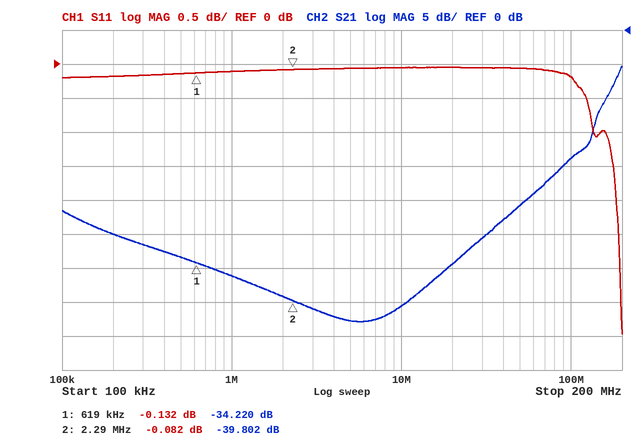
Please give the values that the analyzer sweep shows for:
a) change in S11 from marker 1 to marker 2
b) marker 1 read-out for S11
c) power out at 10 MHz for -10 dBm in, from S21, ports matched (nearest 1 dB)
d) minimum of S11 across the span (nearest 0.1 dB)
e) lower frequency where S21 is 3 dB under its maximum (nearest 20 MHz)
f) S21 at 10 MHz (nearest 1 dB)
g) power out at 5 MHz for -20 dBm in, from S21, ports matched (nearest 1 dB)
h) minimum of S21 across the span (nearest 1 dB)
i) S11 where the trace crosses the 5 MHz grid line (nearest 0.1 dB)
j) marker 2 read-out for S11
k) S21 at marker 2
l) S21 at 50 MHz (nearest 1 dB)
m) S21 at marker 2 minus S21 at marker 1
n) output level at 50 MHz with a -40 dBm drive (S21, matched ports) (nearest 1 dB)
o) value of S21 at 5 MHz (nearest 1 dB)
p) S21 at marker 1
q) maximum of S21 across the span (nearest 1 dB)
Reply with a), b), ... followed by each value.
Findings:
a) 0.050 dB
b) -0.132 dB
c) -51 dBm
d) -4.0 dB
e) 180 MHz
f) -41 dB
g) -63 dBm
h) -43 dB
i) -0.1 dB
j) -0.082 dB
k) -39.802 dB
l) -26 dB
m) -5.582 dB
n) -66 dBm
o) -43 dB
p) -34.220 dB
q) -5 dB
